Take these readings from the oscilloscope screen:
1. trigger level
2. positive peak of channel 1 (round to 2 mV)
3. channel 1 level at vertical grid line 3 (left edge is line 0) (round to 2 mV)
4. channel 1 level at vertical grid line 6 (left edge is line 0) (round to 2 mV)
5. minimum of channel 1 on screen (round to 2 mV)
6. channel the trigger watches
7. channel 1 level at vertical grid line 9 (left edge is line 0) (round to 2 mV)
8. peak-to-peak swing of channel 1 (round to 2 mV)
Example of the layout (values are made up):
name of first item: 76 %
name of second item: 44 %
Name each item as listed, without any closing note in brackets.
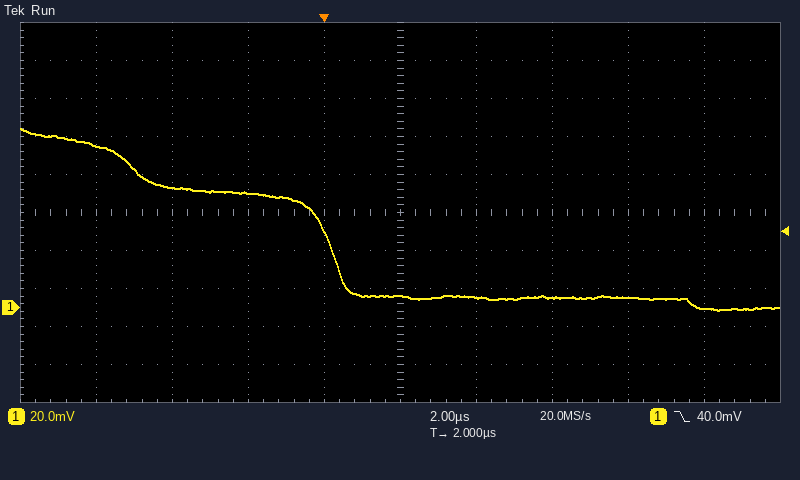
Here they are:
trigger level: 40.0 mV
positive peak of channel 1: 94 mV
channel 1 level at vertical grid line 3 (left edge is line 0): 60 mV
channel 1 level at vertical grid line 6 (left edge is line 0): 6 mV
minimum of channel 1 on screen: -2 mV
channel the trigger watches: channel 1
channel 1 level at vertical grid line 9 (left edge is line 0): 0 mV
peak-to-peak swing of channel 1: 96 mV
